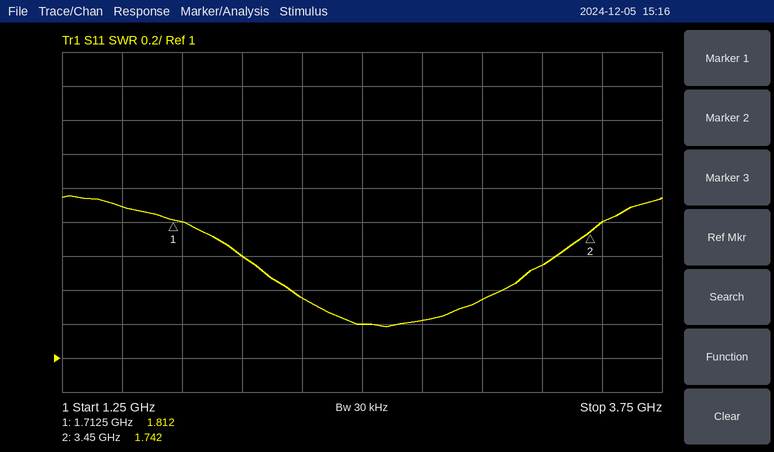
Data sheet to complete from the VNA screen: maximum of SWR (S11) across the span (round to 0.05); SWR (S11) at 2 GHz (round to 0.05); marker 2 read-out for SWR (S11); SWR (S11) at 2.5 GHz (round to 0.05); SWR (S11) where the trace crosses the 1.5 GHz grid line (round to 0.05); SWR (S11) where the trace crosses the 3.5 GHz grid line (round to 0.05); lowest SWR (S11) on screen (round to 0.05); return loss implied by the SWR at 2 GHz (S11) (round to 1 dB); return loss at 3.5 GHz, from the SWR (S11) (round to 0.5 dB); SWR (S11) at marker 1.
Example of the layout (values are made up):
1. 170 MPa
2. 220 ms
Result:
1. 1.95
2. 1.60
3. 1.742
4. 1.20
5. 1.90
6. 1.80
7. 1.20
8. 13 dB
9. 11.0 dB
10. 1.812
